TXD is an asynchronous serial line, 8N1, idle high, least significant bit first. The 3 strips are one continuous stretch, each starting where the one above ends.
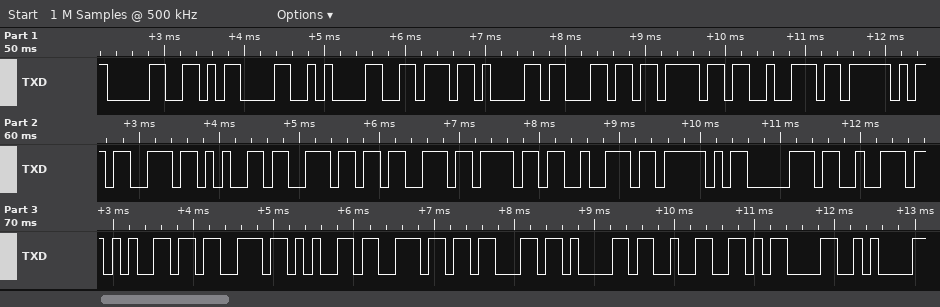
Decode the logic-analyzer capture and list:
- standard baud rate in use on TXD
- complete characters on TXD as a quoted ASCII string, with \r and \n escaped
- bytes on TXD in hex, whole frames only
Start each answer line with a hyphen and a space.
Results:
- 9600 baud
- "0\r\nvalor_sensor_presenca2\r\n"
- 30 0D 0A 76 61 6C 6F 72 5F 73 65 6E 73 6F 72 5F 70 72 65 73 65 6E 63 61 32 0D 0A
